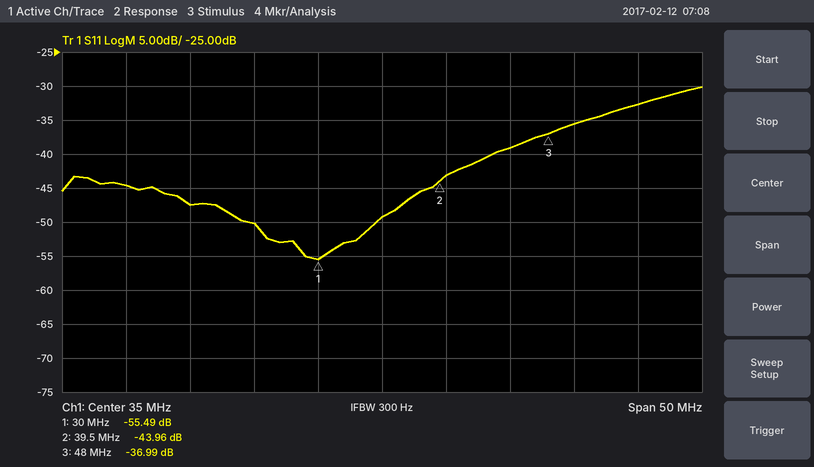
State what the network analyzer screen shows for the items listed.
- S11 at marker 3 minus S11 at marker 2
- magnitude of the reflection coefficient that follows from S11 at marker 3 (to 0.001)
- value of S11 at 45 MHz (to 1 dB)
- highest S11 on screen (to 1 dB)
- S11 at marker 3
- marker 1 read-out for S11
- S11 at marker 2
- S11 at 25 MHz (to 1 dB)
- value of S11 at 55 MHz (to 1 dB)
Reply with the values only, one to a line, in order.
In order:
6.97 dB
0.014
-39 dB
-30 dB
-36.99 dB
-55.49 dB
-43.96 dB
-50 dB
-33 dB
